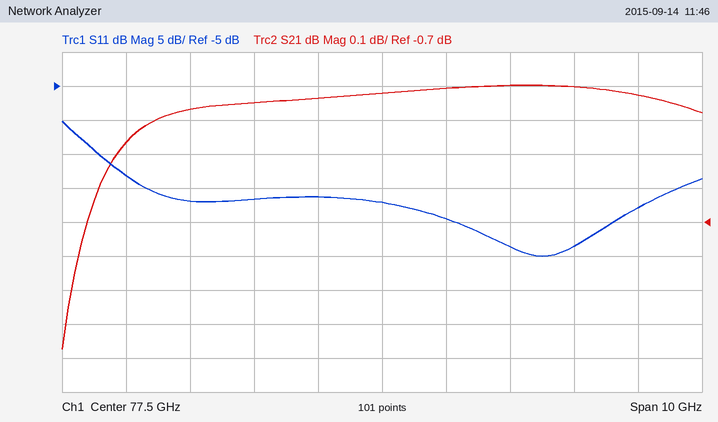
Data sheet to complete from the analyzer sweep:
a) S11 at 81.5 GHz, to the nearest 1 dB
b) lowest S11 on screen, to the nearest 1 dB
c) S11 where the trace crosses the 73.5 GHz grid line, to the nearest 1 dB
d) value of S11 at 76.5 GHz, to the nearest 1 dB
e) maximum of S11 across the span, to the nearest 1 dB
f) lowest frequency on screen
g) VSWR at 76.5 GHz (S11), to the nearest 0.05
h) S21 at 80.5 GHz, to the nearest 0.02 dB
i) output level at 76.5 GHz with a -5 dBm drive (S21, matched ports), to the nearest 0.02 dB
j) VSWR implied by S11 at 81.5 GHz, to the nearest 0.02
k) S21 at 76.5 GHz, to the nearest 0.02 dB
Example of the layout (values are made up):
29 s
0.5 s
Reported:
-23 dB
-30 dB
-18 dB
-21 dB
-10 dB
72.5 GHz
1.20
-0.30 dB
-5.34 dBm
1.16
-0.34 dB
